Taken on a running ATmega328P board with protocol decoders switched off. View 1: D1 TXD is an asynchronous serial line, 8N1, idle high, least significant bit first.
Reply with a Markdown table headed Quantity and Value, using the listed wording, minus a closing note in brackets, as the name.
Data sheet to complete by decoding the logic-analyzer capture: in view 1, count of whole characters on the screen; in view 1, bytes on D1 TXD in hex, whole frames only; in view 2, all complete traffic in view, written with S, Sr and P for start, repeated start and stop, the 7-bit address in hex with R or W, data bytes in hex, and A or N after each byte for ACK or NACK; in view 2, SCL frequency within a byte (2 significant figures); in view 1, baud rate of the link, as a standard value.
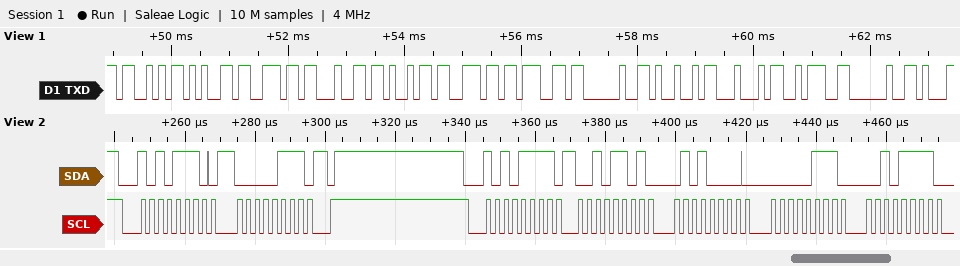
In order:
| Quantity | Value |
|---|---|
| in view 1, count of whole characters on the screen | 12 |
| in view 1, bytes on D1 TXD in hex, whole frames only | 53 65 6E 64 69 6E 67 20 49 44 3A 20 |
| in view 2, all complete traffic in view, written with S, Sr and P for start, repeated start and stop, the 7-bit address in hex with R or W, data bytes in hex, and A or N after each byte for ACK or NACK | S 57W A 07 A P S 57R A 2D A 50 A 07 A 2F A |
| in view 2, SCL frequency within a byte | 400 kHz |
| in view 1, baud rate of the link, as a standard value | 9600 baud |
